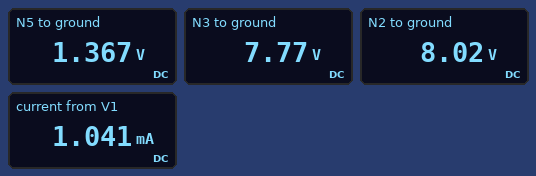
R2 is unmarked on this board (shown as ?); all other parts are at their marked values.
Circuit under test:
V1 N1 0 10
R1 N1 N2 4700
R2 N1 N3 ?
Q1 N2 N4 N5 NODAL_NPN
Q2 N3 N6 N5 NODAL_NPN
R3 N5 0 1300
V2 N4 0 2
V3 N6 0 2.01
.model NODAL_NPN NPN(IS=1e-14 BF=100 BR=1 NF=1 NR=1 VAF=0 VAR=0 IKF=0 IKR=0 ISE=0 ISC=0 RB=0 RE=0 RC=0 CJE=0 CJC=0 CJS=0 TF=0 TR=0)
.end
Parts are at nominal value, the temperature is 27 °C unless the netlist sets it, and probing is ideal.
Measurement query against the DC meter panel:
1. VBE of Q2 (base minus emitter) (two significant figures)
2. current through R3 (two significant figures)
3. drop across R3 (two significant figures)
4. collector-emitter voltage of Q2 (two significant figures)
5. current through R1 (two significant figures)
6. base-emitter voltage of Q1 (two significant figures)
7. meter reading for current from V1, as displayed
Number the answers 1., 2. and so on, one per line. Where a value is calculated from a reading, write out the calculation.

1. 2.01 V - 1.367 V = 640 mV
2. (1.367 V) / 1.3 kΩ = 1.1 mA
3. 1.367 V = 1.4 V
4. 7.77 V - 1.367 V = 6.4 V
5. (10 V - 8.02 V) / 4.7 kΩ = 420 µA
6. 2 V - 1.367 V = 630 mV
7. 1.041 mA
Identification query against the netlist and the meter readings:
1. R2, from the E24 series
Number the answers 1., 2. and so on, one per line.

1. 3.6 kΩ
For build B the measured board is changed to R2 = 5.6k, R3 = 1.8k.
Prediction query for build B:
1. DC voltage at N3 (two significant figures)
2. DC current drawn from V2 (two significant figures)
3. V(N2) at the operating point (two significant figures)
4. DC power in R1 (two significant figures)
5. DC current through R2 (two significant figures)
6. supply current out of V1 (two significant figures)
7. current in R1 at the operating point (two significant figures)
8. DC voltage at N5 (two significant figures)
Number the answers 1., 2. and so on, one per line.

1. 7.5 V
2. 3.1 µA
3. 8.6 V
4. 440 µW
5. 450 µA
6. 760 µA
7. 310 µA
8. 1.4 V
